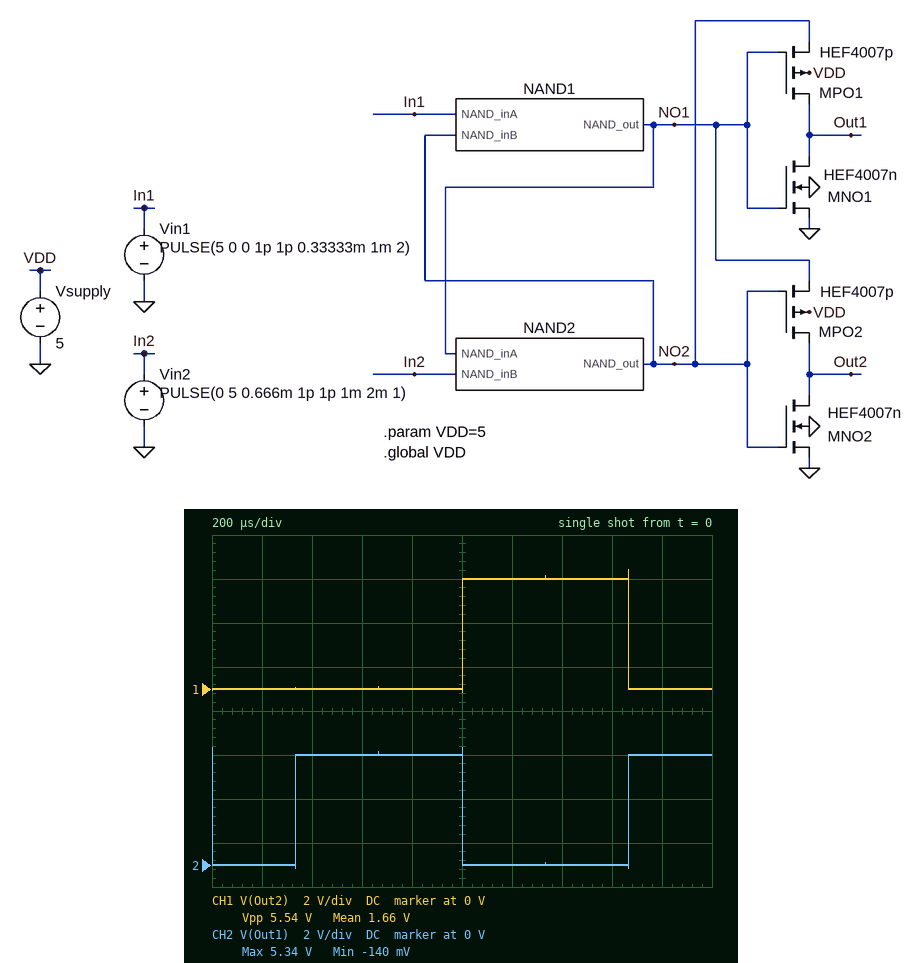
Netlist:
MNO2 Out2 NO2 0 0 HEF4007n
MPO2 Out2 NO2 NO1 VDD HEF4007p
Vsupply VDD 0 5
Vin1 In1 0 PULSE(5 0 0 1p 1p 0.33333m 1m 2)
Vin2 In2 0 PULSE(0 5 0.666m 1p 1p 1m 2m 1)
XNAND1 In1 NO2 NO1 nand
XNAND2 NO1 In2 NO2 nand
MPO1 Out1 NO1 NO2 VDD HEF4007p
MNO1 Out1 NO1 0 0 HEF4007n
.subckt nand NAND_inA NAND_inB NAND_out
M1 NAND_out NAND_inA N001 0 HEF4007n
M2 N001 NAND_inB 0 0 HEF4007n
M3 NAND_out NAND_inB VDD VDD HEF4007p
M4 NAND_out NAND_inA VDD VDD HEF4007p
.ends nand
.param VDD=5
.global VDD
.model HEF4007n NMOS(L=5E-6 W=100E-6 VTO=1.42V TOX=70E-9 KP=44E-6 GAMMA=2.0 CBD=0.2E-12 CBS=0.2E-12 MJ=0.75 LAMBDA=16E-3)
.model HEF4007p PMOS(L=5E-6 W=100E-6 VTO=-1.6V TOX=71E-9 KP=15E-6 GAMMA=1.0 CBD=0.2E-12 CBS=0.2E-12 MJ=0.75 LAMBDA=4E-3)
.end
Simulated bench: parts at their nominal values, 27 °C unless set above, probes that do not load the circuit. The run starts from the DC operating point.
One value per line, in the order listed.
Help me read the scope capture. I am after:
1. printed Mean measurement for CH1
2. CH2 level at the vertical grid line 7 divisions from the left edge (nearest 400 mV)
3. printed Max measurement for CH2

1.66 V
0 V
5.34 V
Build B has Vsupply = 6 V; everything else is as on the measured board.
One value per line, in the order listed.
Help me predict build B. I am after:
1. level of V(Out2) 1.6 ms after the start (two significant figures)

6.0 V
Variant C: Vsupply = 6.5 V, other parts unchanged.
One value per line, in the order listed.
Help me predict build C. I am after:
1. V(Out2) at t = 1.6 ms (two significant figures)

6.5 V
